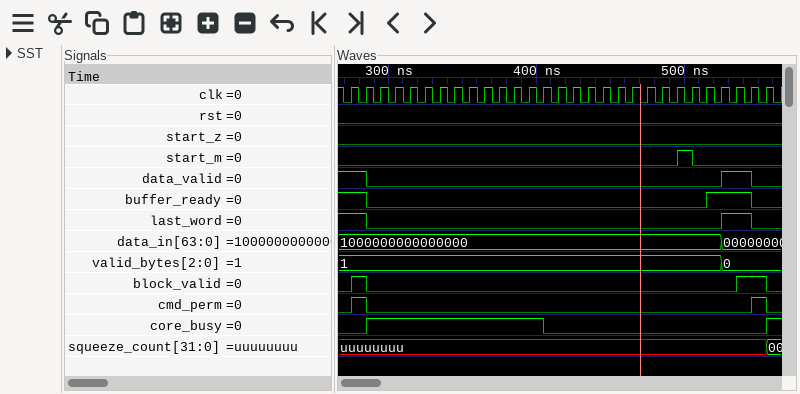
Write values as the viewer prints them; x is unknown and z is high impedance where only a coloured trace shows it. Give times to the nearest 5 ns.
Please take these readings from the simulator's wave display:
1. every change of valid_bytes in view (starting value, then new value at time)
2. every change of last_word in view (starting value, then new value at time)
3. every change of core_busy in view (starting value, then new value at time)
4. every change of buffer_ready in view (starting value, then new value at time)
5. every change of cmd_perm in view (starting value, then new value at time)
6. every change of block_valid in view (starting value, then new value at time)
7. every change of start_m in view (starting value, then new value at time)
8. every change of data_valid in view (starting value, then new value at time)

1, 0 at 525 ns
1, 0 at 285 ns, 1 at 525 ns, 0 at 545 ns
0, 1 at 285 ns, 0 at 405 ns, 1 at 555 ns
1, 0 at 285 ns, 1 at 515 ns, 0 at 545 ns
0, 1 at 275 ns, 0 at 285 ns, 1 at 545 ns, 0 at 555 ns
0, 1 at 275 ns, 0 at 285 ns, 1 at 535 ns, 0 at 555 ns
0, 1 at 495 ns, 0 at 505 ns
1, 0 at 285 ns, 1 at 525 ns, 0 at 545 ns
